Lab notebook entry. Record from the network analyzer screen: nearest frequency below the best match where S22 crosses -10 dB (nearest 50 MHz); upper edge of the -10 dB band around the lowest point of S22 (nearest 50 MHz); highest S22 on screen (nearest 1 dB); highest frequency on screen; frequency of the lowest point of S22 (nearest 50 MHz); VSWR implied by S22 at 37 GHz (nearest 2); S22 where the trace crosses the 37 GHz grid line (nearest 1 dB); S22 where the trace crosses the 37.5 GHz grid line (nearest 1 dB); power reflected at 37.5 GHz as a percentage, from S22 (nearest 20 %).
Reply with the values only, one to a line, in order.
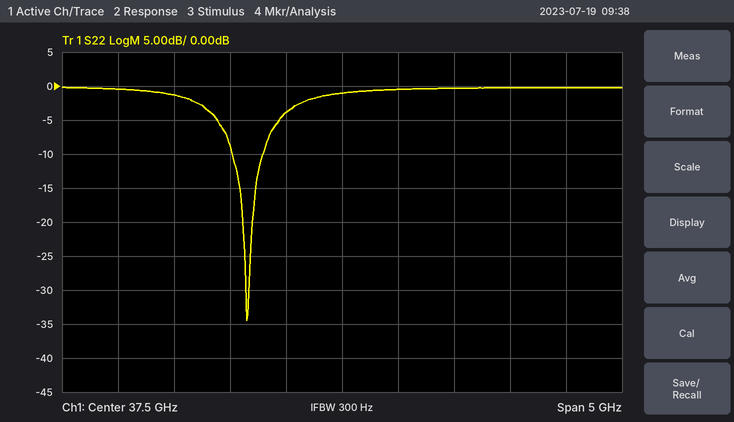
36.50 GHz
36.80 GHz
0 dB
40 GHz
36.65 GHz
4
-4 dB
-1 dB
80 %
